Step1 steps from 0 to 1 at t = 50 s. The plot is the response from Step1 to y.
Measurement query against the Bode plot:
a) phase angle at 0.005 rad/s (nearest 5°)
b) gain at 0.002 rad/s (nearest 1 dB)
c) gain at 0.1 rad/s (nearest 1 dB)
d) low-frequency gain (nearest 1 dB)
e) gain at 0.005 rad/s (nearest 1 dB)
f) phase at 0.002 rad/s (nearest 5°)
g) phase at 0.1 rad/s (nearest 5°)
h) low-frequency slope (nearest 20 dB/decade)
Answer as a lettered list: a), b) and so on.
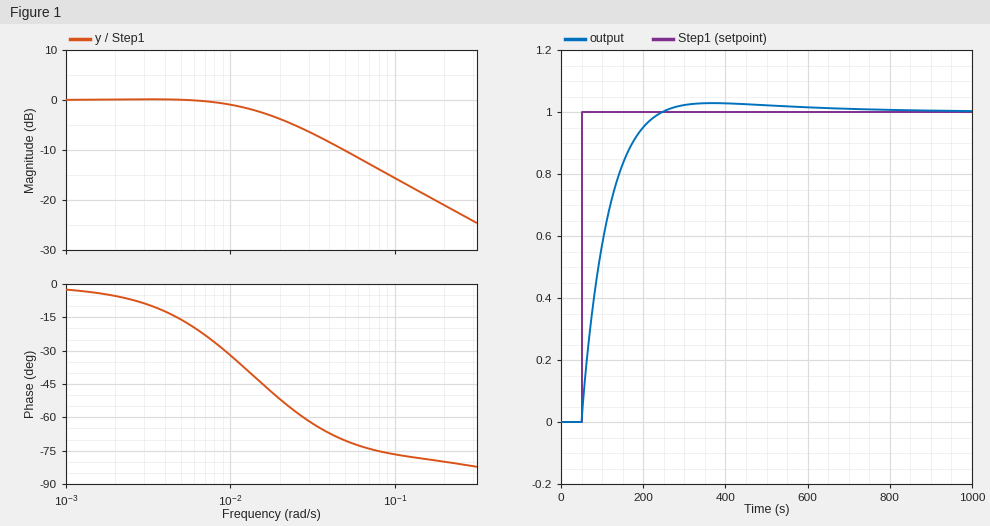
a) -15°
b) 0 dB
c) -16 dB
d) 0 dB
e) 0 dB
f) -5°
g) -75°
h) 0 dB/decade
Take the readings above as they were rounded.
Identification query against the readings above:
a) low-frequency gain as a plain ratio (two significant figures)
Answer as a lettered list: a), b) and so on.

a) 1.0
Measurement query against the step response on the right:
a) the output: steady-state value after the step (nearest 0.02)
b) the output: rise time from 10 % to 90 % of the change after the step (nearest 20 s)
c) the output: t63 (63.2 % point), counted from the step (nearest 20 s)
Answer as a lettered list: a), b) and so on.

a) 1.00
b) 120 s
c) 60 s
